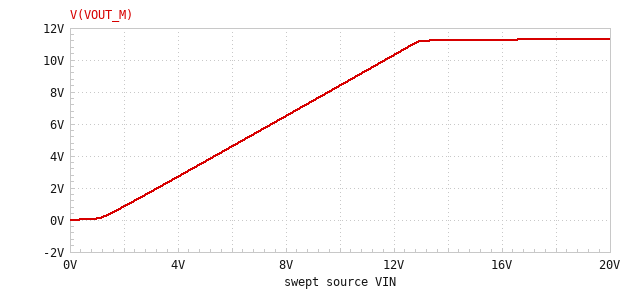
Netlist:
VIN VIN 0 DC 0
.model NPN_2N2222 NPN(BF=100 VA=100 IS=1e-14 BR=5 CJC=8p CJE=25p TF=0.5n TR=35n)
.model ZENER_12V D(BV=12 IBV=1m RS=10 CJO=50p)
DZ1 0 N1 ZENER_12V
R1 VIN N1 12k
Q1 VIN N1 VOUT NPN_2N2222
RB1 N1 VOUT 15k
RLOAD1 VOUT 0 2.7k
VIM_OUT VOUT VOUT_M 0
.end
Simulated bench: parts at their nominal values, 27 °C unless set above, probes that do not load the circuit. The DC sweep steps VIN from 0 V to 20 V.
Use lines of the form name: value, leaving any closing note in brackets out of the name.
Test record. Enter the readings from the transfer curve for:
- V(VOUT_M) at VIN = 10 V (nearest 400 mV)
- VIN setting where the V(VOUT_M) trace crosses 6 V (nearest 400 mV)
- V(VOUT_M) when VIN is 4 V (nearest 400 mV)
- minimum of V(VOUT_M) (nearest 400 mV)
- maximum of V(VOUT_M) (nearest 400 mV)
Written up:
V(VOUT_M) at VIN = 10 V: 8.4 V
VIN setting where the V(VOUT_M) trace crosses 6 V: 7.6 V
V(VOUT_M) when VIN is 4 V: 2.8 V
minimum of V(VOUT_M): 0 V
maximum of V(VOUT_M): 11.2 V
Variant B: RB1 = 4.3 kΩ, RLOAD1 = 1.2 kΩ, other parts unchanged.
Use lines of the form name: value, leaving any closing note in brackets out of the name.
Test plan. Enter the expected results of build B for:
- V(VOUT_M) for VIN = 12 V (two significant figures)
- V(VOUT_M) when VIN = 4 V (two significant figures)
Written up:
V(VOUT_M) for VIN = 12 V: 8.5 V
V(VOUT_M) when VIN = 4 V: 1.4 V
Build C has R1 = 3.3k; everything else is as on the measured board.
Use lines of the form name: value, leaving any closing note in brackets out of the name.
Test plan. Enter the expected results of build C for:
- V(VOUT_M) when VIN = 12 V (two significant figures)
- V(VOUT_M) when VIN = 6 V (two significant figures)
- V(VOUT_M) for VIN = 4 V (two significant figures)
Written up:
V(VOUT_M) when VIN = 12 V: 11 V
V(VOUT_M) when VIN = 6 V: 5.1 V
V(VOUT_M) for VIN = 4 V: 3.2 V
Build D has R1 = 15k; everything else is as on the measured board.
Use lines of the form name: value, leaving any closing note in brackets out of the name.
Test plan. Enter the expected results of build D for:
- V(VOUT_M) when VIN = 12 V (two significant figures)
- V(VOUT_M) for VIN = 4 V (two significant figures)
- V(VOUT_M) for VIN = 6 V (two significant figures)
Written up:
V(VOUT_M) when VIN = 12 V: 10 V
V(VOUT_M) for VIN = 4 V: 2.6 V
V(VOUT_M) for VIN = 6 V: 4.4 V
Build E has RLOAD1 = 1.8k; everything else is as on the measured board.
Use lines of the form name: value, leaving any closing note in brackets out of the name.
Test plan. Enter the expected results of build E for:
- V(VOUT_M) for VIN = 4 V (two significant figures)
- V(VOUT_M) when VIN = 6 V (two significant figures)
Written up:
V(VOUT_M) for VIN = 4 V: 2.6 V
V(VOUT_M) when VIN = 6 V: 4.5 V
